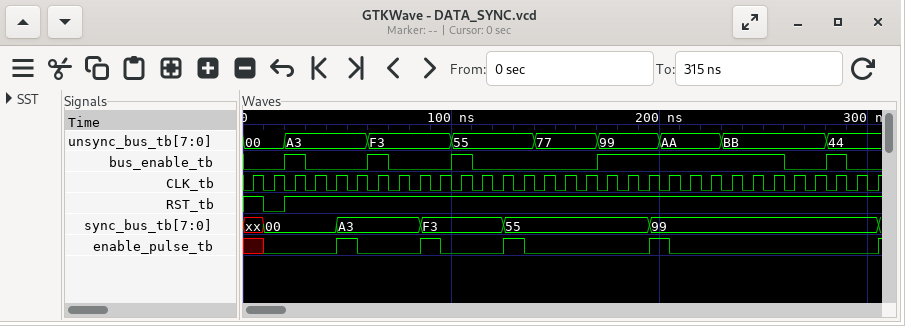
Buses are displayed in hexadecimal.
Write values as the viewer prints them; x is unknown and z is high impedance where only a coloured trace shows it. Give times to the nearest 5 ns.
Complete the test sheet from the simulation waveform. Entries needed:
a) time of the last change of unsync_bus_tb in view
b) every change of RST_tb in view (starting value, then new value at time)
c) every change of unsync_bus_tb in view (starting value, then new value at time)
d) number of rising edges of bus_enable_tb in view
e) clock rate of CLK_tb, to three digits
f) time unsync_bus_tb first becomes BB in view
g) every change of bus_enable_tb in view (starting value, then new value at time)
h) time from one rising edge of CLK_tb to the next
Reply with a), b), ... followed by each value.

a) 280 ns
b) 1, 0 at 10 ns, 1 at 20 ns
c) 00, A3 at 20 ns, F3 at 60 ns, 55 at 100 ns, 77 at 140 ns, 99 at 170 ns, AA at 200 ns, BB at 230 ns, 44 at 280 ns
d) 5
e) 100 MHz
f) 230 ns
g) 0, 1 at 20 ns, 0 at 30 ns, 1 at 60 ns, 0 at 70 ns, 1 at 100 ns, 0 at 110 ns, 1 at 170 ns, 0 at 260 ns, 1 at 280 ns, 0 at 290 ns
h) 10 ns
